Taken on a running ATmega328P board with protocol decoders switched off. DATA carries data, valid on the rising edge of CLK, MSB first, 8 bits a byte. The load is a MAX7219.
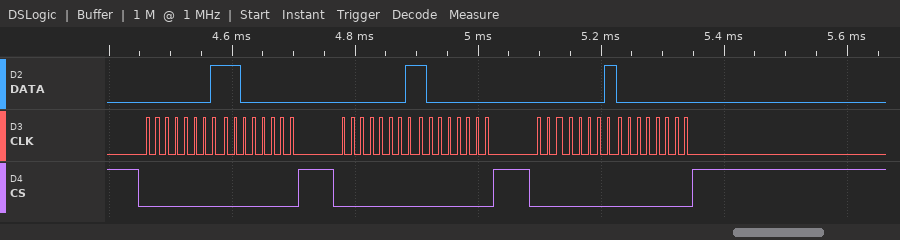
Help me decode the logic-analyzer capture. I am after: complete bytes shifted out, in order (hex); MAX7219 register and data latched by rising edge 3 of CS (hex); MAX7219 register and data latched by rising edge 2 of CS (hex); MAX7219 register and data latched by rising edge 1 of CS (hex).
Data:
0x01 0xC0 0x01 0x80 0x01 0x00
register 0x1, data 0x00
register 0x1, data 0x80
register 0x1, data 0xC0
